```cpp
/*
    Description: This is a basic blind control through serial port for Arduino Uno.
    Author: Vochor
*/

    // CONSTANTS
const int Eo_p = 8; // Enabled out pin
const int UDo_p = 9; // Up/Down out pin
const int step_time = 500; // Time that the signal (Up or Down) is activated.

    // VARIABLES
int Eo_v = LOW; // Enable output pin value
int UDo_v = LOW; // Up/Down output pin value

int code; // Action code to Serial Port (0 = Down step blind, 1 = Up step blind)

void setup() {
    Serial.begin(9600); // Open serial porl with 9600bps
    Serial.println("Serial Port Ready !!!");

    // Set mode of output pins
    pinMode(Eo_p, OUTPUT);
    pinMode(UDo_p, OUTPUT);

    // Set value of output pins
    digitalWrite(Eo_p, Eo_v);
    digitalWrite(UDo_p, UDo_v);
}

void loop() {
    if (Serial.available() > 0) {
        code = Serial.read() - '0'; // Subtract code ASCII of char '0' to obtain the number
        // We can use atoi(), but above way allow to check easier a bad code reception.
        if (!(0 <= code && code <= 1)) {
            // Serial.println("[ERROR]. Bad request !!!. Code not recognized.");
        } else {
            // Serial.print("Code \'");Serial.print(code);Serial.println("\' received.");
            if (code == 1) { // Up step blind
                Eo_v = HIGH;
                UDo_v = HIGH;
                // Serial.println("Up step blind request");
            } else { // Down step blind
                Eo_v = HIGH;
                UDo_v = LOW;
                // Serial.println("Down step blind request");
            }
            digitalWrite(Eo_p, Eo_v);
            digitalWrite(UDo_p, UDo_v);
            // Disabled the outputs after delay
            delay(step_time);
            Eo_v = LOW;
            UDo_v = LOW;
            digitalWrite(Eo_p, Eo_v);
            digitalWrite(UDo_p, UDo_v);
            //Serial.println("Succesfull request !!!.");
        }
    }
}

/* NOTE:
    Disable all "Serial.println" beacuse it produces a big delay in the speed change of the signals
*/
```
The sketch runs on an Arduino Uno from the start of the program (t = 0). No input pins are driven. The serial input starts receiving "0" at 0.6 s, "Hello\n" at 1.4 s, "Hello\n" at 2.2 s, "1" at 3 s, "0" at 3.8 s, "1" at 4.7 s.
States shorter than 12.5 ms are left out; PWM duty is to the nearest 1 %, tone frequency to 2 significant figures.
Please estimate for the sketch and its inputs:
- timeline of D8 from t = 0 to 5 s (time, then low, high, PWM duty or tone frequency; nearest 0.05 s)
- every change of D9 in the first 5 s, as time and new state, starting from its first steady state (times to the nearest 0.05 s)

0 s low; 0.6 s high; 1.1 s low; 3 s high; 3.5 s low; 3.8 s high; 4.3 s low; 4.7 s high
0 s low; 3 s high; 3.5 s low; 4.7 s high
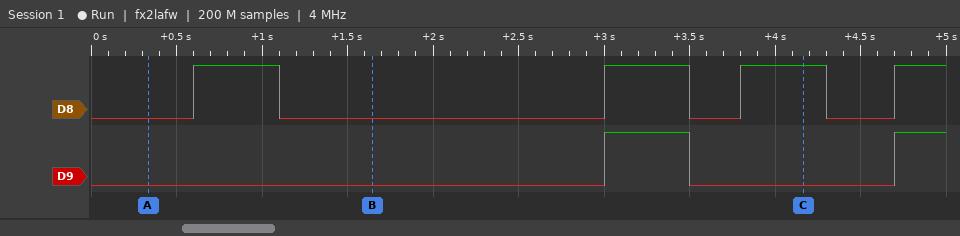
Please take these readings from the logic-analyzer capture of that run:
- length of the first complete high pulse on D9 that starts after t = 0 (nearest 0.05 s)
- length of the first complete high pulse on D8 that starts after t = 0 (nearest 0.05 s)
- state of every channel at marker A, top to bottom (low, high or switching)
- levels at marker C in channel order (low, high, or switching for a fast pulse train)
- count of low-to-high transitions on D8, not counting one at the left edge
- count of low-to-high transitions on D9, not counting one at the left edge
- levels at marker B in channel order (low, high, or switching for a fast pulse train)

0.50 s
0.50 s
D8 low, D9 low
D8 high, D9 low
4
2
D8 low, D9 low
